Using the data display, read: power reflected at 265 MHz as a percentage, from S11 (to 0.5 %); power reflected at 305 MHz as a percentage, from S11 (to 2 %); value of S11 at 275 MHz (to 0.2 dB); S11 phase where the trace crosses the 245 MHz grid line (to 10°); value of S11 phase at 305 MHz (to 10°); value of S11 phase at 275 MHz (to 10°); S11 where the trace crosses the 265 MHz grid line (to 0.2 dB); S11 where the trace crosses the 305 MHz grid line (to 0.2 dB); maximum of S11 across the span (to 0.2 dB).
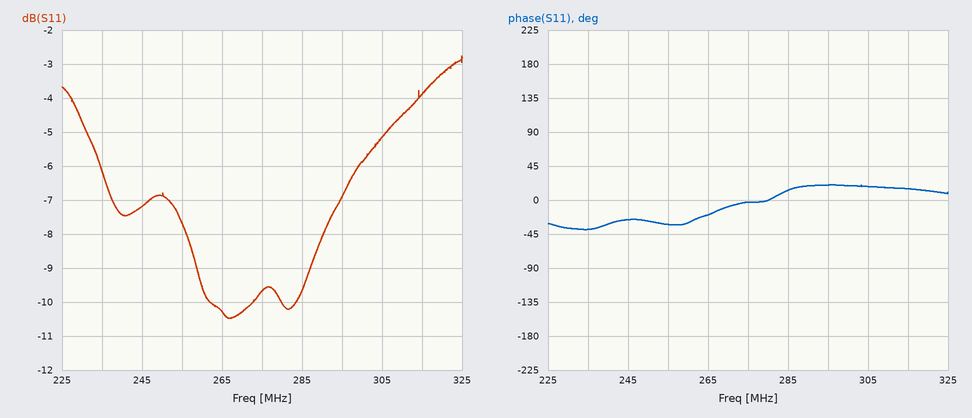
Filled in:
9.5 %
30 %
-9.6 dB
-30°
20°
0°
-10.2 dB
-5.2 dB
-2.8 dB
